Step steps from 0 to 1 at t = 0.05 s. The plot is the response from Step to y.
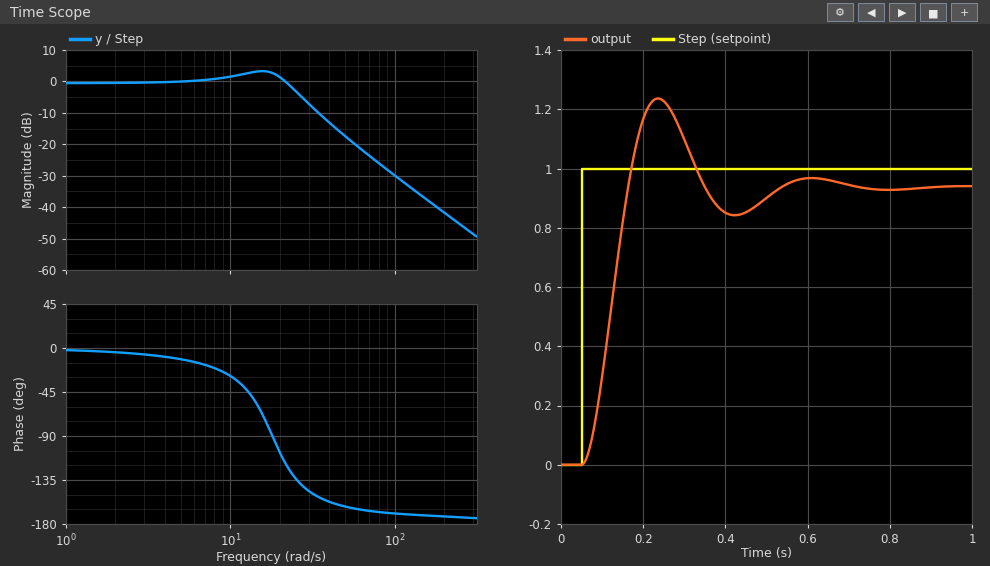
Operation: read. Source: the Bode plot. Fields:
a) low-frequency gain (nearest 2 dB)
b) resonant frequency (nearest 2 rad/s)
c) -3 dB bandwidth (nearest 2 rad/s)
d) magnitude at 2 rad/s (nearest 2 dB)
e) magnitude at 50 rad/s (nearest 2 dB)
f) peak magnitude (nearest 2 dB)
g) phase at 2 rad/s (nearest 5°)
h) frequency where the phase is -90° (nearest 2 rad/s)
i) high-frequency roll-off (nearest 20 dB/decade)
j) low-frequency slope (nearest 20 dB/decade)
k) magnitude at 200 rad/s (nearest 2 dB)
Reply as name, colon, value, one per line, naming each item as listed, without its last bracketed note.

low-frequency gain: 0 dB
resonant frequency: 16 rad/s
-3 dB bandwidth: 26 rad/s
magnitude at 2 rad/s: 0 dB
magnitude at 50 rad/s: -18 dB
peak magnitude: 4 dB
phase at 2 rad/s: -5°
frequency where the phase is -90°: 18 rad/s
high-frequency roll-off: -40 dB/decade
low-frequency slope: 0 dB/decade
magnitude at 200 rad/s: -42 dB
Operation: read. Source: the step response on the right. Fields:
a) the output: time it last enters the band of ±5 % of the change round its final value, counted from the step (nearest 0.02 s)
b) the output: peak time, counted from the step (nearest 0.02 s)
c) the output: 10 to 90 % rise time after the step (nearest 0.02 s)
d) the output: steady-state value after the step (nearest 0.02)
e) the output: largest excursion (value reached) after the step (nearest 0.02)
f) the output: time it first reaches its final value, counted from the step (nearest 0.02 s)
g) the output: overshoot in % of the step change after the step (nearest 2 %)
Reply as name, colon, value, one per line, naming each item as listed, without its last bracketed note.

the output: time it last enters the band of ±5 % of the change round its final value, counted from the step: 0.44 s
the output: peak time, counted from the step: 0.18 s
the output: 10 to 90 % rise time after the step: 0.08 s
the output: steady-state value after the step: 0.94
the output: largest excursion (value reached) after the step: 1.24
the output: time it first reaches its final value, counted from the step: 0.12 s
the output: overshoot in % of the step change after the step: 32 %
